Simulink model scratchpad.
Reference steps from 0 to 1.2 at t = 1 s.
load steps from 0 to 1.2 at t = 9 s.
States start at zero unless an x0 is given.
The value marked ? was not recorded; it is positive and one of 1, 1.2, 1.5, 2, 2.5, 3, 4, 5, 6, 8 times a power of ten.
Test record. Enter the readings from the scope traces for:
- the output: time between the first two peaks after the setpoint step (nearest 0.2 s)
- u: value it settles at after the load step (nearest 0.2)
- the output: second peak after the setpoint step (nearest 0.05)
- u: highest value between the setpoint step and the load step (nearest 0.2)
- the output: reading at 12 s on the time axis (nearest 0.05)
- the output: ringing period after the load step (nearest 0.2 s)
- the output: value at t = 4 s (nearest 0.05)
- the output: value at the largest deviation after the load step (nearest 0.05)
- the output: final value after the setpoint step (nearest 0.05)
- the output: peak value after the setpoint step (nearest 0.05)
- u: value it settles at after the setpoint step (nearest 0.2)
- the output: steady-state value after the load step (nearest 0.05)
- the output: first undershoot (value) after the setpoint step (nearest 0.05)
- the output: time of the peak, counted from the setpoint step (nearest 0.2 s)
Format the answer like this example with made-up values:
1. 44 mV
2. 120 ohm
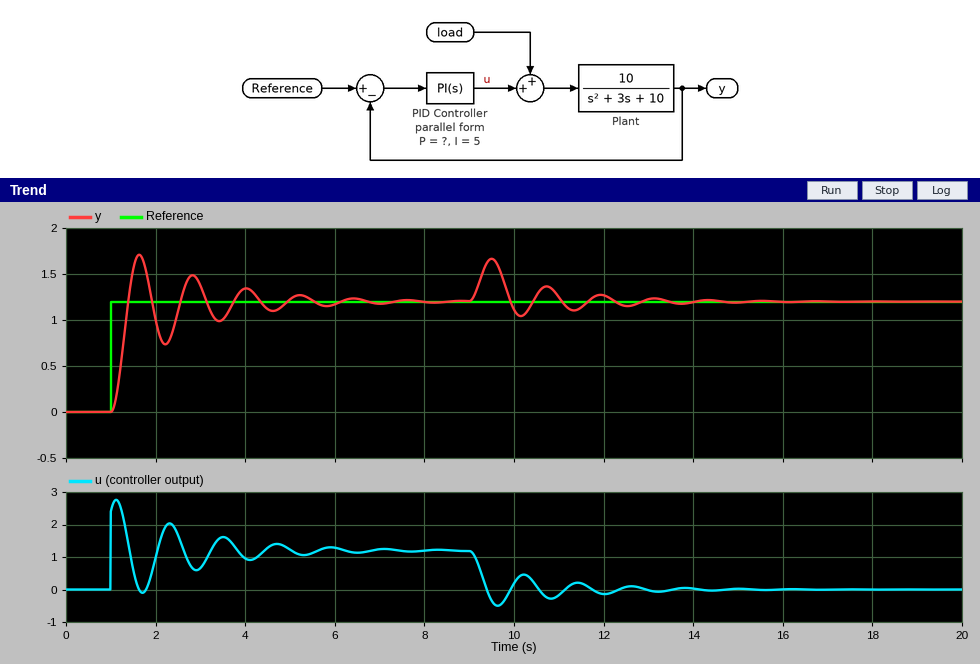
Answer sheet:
1. 1.2 s
2. 0.0
3. 1.50
4. 2.8
5. 1.25
6. 1.2 s
7. 1.35
8. 1.65
9. 1.20
10. 1.70
11. 1.2
12. 1.20
13. 0.75
14. 0.6 s
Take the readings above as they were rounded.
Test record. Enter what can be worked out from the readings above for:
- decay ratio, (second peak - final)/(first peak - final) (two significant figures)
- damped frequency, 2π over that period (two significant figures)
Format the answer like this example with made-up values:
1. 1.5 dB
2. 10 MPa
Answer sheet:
1. 0.60
2. 5.2 rad/s
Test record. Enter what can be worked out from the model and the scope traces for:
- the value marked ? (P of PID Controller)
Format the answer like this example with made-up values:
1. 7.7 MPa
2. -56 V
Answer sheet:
1. 2
